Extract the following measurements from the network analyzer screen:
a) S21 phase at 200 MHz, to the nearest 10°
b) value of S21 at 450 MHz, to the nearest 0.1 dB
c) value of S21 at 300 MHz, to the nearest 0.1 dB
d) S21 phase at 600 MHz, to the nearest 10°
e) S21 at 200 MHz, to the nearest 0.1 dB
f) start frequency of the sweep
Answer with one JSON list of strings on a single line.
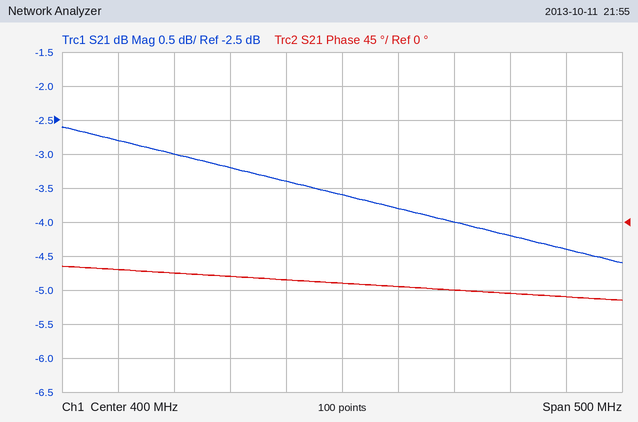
["-60°", "-3.8 dB", "-3.2 dB", "-100°", "-2.8 dB", "150 MHz"]
